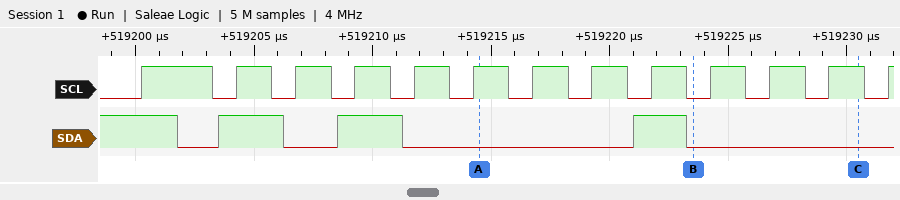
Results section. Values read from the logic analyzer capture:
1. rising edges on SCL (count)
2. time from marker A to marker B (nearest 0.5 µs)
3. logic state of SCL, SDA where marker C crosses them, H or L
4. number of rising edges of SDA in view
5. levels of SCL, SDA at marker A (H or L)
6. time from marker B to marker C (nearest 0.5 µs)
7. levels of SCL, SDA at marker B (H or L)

13
9 µs
SCL=H, SDA=L
3
SCL=H, SDA=L
7 µs
SCL=L, SDA=L
